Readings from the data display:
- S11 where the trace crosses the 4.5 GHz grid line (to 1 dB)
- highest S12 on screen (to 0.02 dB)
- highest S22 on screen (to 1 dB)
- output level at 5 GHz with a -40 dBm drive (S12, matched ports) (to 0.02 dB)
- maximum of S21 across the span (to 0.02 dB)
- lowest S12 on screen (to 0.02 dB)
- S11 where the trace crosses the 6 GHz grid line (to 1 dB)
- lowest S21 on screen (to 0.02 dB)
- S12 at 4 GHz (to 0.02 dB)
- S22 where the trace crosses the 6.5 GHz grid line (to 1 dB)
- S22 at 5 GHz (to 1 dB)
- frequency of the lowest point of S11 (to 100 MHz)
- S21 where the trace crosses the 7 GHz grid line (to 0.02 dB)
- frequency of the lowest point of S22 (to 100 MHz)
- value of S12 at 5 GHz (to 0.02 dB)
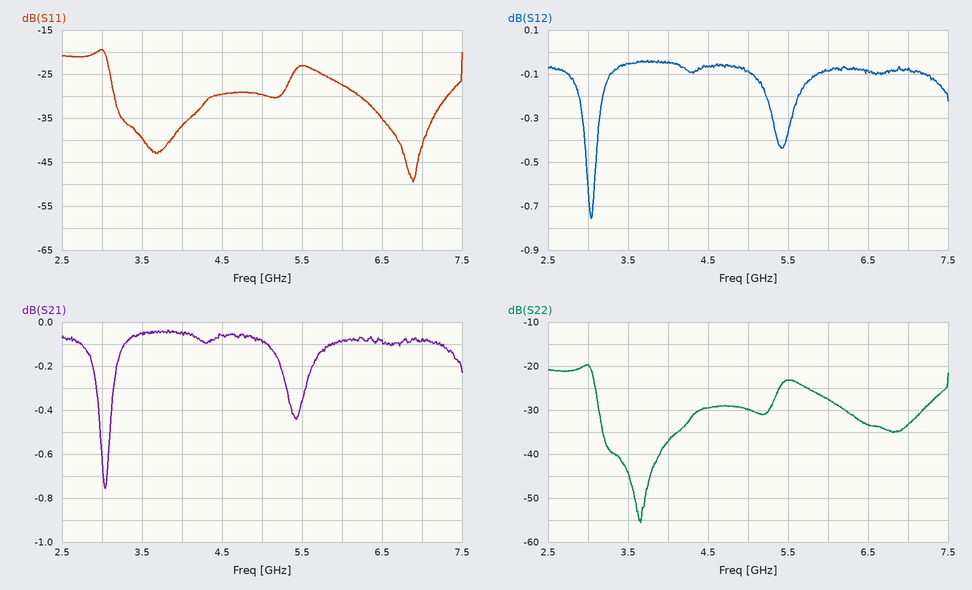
-30 dB
-0.04 dB
-20 dB
-40.08 dBm
-0.04 dB
-0.76 dB
-27 dB
-0.76 dB
-0.04 dB
-33 dB
-30 dB
6.9 GHz
-0.08 dB
3.7 GHz
-0.08 dB
